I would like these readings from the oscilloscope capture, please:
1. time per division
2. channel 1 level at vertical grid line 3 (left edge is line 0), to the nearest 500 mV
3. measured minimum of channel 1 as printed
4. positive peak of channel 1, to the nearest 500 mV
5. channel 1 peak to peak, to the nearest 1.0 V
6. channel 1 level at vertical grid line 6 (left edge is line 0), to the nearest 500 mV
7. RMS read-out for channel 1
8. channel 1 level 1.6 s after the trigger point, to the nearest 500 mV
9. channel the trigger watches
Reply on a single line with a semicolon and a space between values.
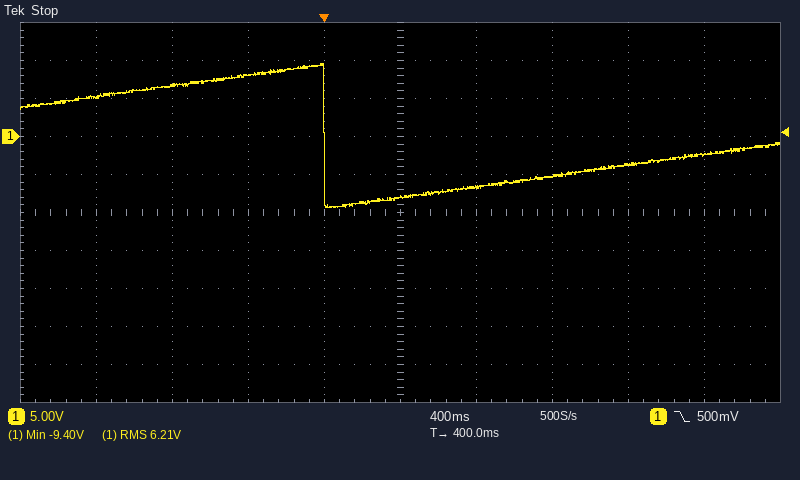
400 ms; 8.0 V; -9.40 V; 9.5 V; 19.0 V; -6.5 V; 6.21 V; -3.5 V; channel 1
